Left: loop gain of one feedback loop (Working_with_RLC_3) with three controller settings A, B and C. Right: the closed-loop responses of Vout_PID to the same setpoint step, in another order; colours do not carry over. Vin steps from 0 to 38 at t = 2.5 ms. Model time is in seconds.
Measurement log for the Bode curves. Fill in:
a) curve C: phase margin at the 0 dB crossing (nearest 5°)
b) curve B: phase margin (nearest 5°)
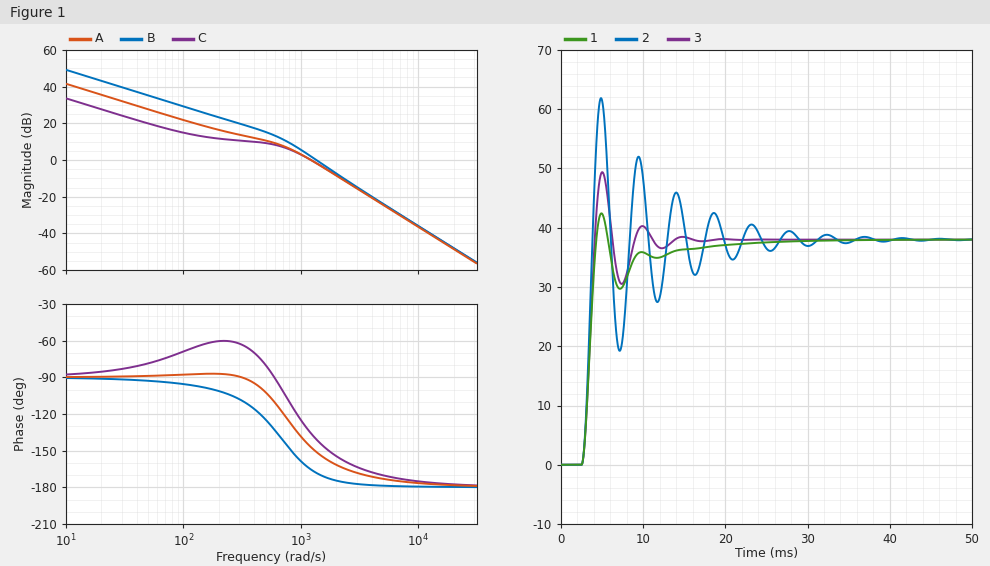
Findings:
45°
10°
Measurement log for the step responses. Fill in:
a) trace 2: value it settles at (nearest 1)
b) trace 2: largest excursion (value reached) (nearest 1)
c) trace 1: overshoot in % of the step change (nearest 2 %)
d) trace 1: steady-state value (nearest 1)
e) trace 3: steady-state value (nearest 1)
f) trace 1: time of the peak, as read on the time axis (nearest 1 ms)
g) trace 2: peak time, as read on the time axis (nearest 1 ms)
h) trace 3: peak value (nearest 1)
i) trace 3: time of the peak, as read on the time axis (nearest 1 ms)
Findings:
38
62
12 %
38
38
5 ms
5 ms
49
5 ms
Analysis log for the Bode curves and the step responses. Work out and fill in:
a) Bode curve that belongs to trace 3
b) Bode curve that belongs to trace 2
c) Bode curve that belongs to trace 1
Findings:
A
B
C
